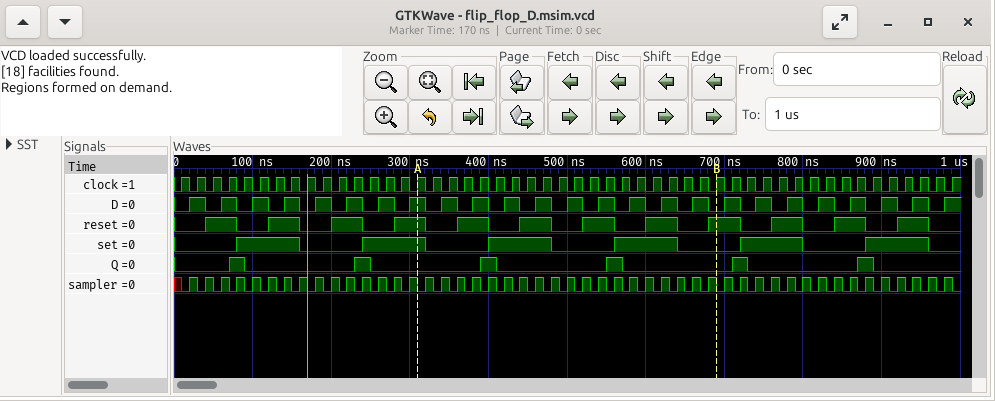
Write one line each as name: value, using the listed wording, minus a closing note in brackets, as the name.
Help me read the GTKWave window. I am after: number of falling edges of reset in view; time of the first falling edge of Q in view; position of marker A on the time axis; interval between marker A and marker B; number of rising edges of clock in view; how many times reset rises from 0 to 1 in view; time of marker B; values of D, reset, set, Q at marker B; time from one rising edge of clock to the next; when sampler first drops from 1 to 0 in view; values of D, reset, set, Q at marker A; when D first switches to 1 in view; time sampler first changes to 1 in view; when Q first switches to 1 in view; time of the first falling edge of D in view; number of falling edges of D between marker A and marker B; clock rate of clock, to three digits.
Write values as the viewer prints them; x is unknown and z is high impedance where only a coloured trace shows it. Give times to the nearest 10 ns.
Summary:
number of falling edges of reset in view: 12
time of the first falling edge of Q in view: 90 ns
position of marker A on the time axis: 310 ns
interval between marker A and marker B: 380 ns
number of rising edges of clock in view: 50
how many times reset rises from 0 to 1 in view: 12
time of marker B: 690 ns
values of D, reset, set, Q at marker B: D=0, reset=1, set=0, Q=0
time from one rising edge of clock to the next: 20 ns
when sampler first drops from 1 to 0 in view: 30 ns
values of D, reset, set, Q at marker A: D=1, reset=1, set=1, Q=0
when D first switches to 1 in view: 20 ns
time sampler first changes to 1 in view: 20 ns
when Q first switches to 1 in view: 70 ns
time of the first falling edge of D in view: 40 ns
number of falling edges of D between marker A and marker B: 10
clock rate of clock, to three digits: 50.0 MHz
